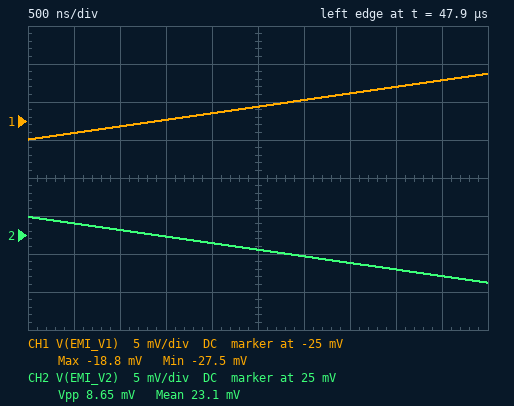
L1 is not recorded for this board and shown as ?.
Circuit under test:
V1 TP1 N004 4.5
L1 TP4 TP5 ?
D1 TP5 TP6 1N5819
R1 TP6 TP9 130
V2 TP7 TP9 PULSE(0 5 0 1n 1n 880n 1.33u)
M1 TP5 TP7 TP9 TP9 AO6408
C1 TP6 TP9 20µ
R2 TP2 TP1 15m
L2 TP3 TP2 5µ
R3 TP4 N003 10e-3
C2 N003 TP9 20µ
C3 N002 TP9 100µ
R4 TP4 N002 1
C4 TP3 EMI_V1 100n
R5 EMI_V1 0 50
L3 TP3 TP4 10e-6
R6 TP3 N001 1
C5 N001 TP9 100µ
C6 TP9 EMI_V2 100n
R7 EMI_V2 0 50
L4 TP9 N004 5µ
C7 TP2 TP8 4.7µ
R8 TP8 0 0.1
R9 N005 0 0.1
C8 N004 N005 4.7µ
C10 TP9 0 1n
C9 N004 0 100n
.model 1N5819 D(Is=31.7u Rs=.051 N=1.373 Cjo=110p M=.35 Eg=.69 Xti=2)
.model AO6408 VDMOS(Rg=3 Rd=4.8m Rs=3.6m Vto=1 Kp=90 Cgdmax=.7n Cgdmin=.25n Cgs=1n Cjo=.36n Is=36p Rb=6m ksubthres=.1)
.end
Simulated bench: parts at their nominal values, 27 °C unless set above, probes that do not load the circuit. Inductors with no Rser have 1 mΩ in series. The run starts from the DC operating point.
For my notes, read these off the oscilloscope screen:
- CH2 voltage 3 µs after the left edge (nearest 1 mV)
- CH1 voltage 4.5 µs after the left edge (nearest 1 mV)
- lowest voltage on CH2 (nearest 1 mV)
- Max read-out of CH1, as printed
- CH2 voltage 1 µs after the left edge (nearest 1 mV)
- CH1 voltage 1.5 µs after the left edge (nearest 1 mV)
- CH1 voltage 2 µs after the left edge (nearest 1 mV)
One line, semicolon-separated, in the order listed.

22 mV; -20 mV; 19 mV; -18.8 mV; 26 mV; -25 mV; -24 mV
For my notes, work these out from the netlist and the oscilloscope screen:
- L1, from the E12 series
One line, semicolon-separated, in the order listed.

33 µH
